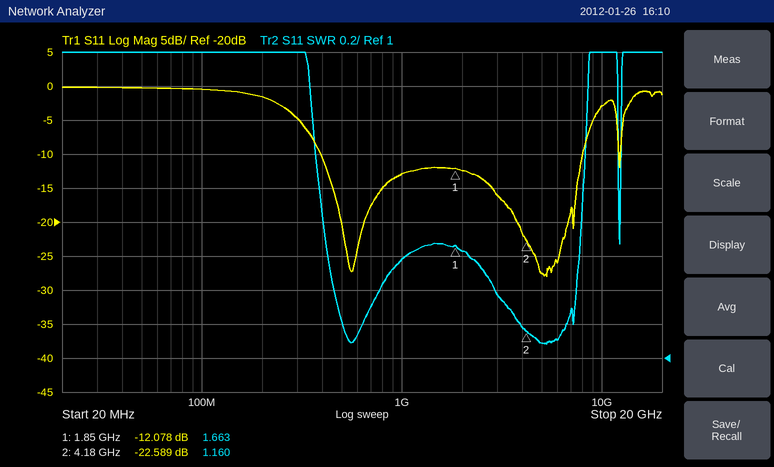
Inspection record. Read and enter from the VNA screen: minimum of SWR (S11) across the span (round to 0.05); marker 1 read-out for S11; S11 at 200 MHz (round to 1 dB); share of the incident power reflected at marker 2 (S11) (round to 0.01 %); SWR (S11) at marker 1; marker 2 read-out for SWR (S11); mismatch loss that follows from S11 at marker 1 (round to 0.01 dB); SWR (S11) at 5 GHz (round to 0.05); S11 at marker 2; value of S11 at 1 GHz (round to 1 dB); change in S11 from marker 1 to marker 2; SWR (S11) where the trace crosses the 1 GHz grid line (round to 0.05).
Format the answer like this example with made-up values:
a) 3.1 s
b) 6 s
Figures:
a) 1.10
b) -12.078 dB
c) -2 dB
d) 0.55 %
e) 1.663
f) 1.160
g) 0.28 dB
h) 1.10
i) -22.589 dB
j) -13 dB
k) -10.511 dB
l) 1.60
